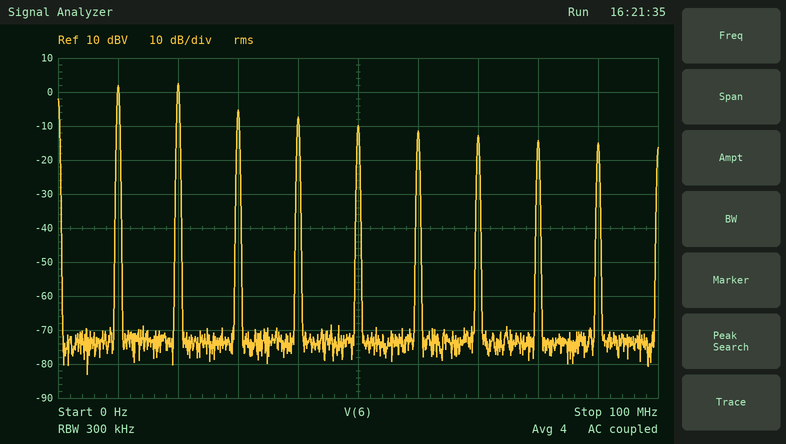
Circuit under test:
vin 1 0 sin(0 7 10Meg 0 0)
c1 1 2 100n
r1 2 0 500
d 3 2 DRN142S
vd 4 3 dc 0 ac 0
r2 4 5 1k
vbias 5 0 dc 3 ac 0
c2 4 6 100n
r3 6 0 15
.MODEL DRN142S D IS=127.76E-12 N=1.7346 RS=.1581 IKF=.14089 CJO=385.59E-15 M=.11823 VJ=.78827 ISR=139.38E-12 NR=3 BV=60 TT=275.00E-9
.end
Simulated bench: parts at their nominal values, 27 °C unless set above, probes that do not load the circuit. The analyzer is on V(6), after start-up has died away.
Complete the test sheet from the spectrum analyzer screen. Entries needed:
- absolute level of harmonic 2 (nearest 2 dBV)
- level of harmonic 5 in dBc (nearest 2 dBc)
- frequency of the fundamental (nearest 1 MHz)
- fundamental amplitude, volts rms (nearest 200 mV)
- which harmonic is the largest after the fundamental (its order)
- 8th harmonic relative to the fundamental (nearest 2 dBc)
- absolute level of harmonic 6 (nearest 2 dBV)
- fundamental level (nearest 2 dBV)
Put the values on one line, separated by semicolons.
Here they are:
2 dBV; -12 dBc; 10 MHz; 1.2 V; 2; -16 dBc; -12 dBV; 2 dBV
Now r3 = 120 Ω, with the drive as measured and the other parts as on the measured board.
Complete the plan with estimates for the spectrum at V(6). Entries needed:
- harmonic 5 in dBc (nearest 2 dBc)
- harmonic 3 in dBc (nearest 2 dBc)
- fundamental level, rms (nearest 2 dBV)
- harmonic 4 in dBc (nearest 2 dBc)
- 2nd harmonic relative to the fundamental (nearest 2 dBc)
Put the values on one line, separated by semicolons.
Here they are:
-22 dBc; -14 dBc; 12 dBV; -18 dBc; -10 dBc
